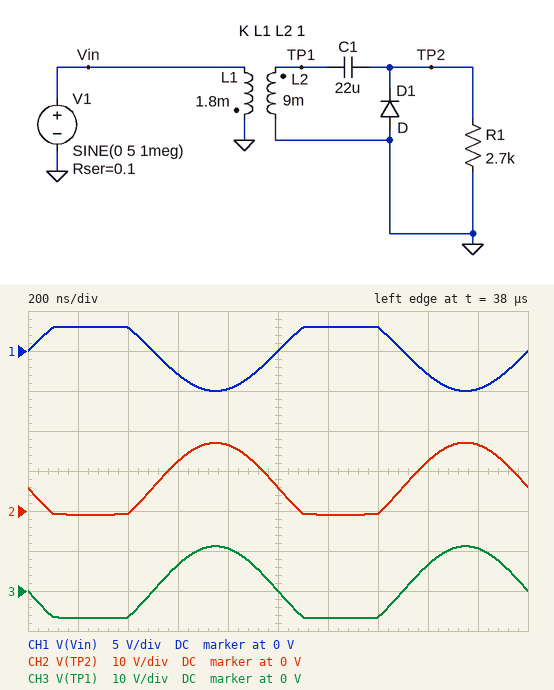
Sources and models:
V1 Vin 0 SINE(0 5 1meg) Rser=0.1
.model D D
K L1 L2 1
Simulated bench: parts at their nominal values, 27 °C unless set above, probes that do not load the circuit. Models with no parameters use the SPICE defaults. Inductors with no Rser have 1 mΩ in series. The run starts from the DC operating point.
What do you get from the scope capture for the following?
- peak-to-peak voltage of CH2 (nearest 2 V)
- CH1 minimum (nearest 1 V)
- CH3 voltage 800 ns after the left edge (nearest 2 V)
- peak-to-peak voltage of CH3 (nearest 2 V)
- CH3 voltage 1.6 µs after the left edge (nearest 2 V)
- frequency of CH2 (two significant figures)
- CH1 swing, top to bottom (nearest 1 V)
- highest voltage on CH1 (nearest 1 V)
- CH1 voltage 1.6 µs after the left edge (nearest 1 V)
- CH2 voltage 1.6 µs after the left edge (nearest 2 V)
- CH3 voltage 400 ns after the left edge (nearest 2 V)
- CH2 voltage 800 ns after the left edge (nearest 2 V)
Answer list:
18 V
-5 V
10 V
18 V
6 V
1.0 MHz
8 V
3 V
-3 V
12 V
-6 V
16 V
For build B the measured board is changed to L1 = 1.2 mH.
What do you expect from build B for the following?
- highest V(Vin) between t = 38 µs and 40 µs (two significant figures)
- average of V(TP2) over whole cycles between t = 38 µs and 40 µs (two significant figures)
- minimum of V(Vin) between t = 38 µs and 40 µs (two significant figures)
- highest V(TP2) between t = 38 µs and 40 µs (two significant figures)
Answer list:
2.5 V
7.4 V
-5.0 V
20 V
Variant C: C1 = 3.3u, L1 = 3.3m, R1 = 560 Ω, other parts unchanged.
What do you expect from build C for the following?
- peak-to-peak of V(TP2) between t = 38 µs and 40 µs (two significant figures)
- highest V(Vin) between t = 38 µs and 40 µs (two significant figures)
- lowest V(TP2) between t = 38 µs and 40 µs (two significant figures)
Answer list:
16 V
4.9 V
-820 mV
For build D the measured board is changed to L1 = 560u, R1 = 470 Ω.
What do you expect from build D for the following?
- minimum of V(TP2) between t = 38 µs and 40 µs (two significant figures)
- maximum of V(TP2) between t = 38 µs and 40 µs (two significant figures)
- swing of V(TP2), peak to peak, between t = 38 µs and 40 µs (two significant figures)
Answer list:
-890 mV
25 V
26 V
